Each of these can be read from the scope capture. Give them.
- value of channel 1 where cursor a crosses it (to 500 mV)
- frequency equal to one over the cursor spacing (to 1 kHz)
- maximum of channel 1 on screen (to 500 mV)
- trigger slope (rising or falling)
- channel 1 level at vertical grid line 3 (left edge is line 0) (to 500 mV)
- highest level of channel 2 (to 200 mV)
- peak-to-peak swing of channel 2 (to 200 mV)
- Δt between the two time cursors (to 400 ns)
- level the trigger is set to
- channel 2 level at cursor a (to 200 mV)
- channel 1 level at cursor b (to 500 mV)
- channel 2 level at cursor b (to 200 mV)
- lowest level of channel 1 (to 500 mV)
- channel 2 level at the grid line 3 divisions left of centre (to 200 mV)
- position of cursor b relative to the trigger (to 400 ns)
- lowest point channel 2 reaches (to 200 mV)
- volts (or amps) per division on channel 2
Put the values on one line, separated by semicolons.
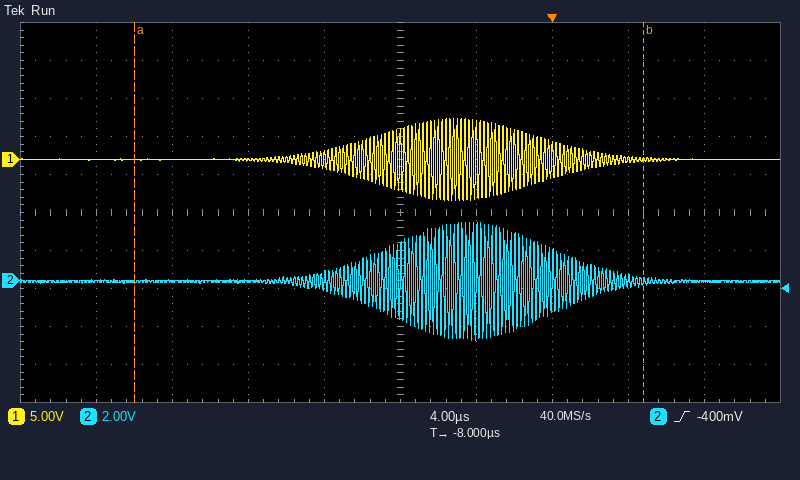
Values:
0.0 V; 37 kHz; 5.5 V; rising; 0.0 V; 3.0 V; 6.2 V; 26.8 µs; -400 mV; 0.0 V; 0.0 V; 0.0 V; -5.5 V; 0.0 V; +4.8 µs; -3.2 V; 2 V
